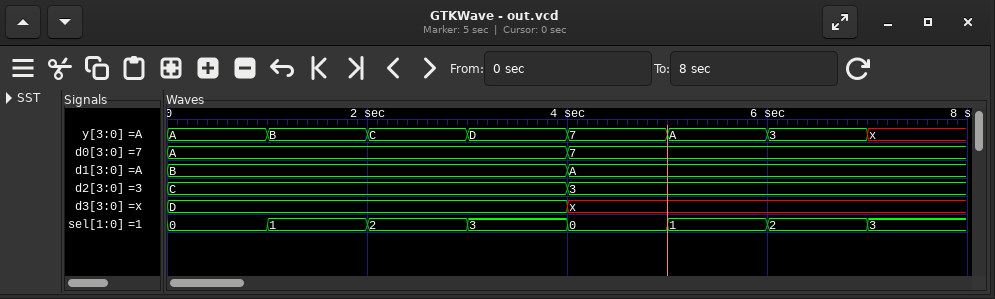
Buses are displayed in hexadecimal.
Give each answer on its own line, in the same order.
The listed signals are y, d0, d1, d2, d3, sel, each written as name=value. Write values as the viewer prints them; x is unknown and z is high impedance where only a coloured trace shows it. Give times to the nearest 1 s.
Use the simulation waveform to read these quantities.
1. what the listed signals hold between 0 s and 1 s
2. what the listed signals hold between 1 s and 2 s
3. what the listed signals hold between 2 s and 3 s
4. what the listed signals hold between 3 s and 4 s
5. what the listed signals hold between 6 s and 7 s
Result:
y=A, d0=A, d1=B, d2=C, d3=D, sel=0
y=B, d0=A, d1=B, d2=C, d3=D, sel=1
y=C, d0=A, d1=B, d2=C, d3=D, sel=2
y=D, d0=A, d1=B, d2=C, d3=D, sel=3
y=3, d0=7, d1=A, d2=3, d3=x, sel=2
